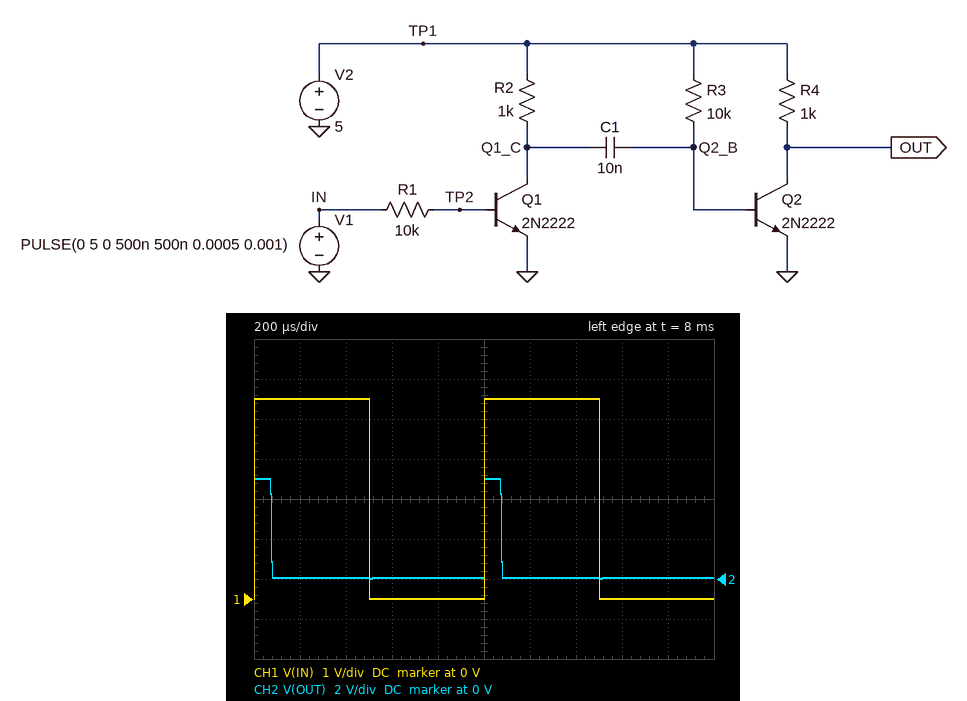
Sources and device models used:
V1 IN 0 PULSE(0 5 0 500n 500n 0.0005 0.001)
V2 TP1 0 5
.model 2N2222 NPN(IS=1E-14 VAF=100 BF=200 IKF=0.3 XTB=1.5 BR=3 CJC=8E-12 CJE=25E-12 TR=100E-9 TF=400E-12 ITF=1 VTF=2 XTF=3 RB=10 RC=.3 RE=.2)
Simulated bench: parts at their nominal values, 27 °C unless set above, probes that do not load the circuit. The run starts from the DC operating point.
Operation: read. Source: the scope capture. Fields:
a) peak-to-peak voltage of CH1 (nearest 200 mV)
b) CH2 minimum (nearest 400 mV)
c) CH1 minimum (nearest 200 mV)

5.0 V
0 V
0 V
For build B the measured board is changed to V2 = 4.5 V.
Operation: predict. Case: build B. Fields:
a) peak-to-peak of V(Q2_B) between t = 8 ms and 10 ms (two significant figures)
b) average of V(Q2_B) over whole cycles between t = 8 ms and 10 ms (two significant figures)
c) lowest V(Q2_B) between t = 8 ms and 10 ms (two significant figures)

4.5 V
560 mV
-3.7 V
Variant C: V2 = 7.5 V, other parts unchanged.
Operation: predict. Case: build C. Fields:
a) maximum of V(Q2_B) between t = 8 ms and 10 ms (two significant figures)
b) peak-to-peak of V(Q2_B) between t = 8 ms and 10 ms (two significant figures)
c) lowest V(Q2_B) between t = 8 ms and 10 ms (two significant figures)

830 mV
7.4 V
-6.6 V
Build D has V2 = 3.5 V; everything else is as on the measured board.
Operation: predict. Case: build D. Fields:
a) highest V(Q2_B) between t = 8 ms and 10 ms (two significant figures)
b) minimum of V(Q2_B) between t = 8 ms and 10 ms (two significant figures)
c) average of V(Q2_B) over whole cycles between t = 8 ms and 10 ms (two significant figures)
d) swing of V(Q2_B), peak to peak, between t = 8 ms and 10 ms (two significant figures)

760 mV
-2.7 V
580 mV
3.5 V
